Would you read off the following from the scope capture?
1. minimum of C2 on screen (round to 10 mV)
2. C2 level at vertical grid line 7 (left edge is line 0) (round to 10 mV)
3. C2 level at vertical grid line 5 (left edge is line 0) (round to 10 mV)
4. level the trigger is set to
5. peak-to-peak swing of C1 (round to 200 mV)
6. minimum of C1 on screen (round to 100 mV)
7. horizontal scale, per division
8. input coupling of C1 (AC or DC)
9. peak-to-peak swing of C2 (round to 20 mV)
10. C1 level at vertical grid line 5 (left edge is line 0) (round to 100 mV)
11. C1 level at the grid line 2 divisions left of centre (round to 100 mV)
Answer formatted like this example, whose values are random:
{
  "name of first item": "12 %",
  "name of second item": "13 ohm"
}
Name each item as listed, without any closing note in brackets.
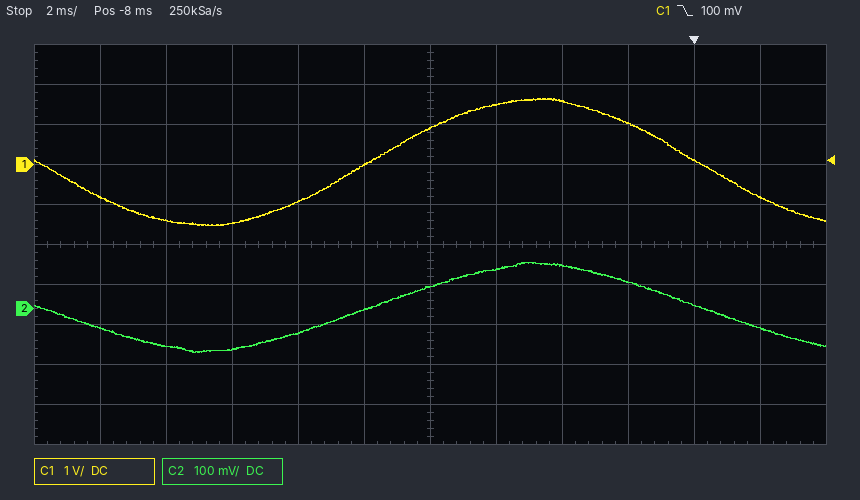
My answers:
{
  "minimum of C2 on screen": "-110 mV",
  "C2 level at vertical grid line 7 (left edge is line 0)": "100 mV",
  "C2 level at vertical grid line 5 (left edge is line 0)": "0 mV",
  "level the trigger is set to": "100 mV",
  "peak-to-peak swing of C1": "3.2 V",
  "minimum of C1 on screen": "-1.5 V",
  "horizontal scale, per division": "2 ms",
  "input coupling of C1": "DC",
  "peak-to-peak swing of C2": "220 mV",
  "C1 level at vertical grid line 5 (left edge is line 0)": "0.0 V",
  "C1 level at the grid line 2 divisions left of centre": "-900 mV"
}
